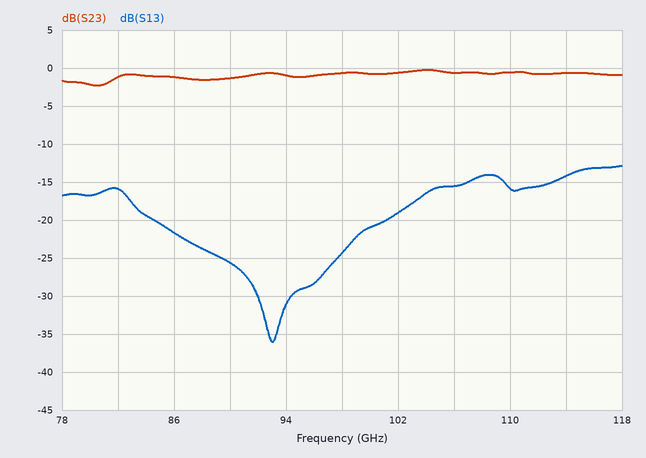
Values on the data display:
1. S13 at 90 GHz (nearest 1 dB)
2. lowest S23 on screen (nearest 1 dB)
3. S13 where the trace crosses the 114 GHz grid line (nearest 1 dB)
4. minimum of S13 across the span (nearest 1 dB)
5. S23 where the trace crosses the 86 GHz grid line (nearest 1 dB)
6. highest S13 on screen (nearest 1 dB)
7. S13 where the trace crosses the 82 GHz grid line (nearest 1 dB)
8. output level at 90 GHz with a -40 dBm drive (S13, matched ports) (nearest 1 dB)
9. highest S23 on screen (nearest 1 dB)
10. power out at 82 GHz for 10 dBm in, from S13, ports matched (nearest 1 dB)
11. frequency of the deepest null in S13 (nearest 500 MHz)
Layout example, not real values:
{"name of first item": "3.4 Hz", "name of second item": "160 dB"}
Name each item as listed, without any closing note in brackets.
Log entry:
{"S13 at 90 GHz": "-26 dB", "lowest S23 on screen": "-2 dB", "S13 where the trace crosses the 114 GHz grid line": "-14 dB", "minimum of S13 across the span": "-36 dB", "S23 where the trace crosses the 86 GHz grid line": "-1 dB", "highest S13 on screen": "-13 dB", "S13 where the trace crosses the 82 GHz grid line": "-16 dB", "output level at 90 GHz with a -40 dBm drive (S13, matched ports)": "-66 dBm", "highest S23 on screen": "0 dB", "power out at 82 GHz for 10 dBm in, from S13, ports matched": "-6 dBm", "frequency of the deepest null in S13": "93.0 GHz"}
